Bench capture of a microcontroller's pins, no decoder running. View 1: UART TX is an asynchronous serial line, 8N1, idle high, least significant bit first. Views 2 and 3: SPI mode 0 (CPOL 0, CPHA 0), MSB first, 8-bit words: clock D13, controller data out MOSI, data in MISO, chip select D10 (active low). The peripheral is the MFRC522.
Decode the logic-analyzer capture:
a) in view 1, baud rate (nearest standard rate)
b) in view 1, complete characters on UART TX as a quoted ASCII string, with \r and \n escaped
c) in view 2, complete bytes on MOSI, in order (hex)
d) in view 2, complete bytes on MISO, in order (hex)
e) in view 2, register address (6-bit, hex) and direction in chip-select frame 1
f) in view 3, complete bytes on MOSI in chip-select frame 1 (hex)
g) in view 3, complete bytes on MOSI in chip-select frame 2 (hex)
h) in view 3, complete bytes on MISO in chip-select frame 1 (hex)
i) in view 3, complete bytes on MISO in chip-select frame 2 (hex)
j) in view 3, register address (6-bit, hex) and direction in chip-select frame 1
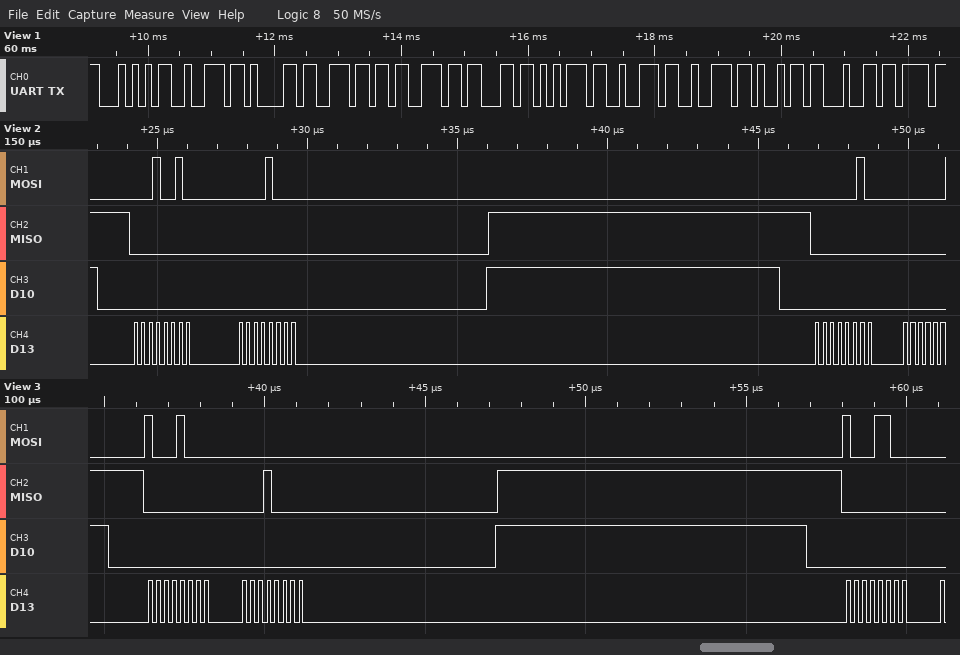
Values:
9600 baud
"Transcurrid"
12 08 02
00 00 00
0x09 write
0x88 0x00
0x8C
0x00 0x10
0x00
0x04 read
